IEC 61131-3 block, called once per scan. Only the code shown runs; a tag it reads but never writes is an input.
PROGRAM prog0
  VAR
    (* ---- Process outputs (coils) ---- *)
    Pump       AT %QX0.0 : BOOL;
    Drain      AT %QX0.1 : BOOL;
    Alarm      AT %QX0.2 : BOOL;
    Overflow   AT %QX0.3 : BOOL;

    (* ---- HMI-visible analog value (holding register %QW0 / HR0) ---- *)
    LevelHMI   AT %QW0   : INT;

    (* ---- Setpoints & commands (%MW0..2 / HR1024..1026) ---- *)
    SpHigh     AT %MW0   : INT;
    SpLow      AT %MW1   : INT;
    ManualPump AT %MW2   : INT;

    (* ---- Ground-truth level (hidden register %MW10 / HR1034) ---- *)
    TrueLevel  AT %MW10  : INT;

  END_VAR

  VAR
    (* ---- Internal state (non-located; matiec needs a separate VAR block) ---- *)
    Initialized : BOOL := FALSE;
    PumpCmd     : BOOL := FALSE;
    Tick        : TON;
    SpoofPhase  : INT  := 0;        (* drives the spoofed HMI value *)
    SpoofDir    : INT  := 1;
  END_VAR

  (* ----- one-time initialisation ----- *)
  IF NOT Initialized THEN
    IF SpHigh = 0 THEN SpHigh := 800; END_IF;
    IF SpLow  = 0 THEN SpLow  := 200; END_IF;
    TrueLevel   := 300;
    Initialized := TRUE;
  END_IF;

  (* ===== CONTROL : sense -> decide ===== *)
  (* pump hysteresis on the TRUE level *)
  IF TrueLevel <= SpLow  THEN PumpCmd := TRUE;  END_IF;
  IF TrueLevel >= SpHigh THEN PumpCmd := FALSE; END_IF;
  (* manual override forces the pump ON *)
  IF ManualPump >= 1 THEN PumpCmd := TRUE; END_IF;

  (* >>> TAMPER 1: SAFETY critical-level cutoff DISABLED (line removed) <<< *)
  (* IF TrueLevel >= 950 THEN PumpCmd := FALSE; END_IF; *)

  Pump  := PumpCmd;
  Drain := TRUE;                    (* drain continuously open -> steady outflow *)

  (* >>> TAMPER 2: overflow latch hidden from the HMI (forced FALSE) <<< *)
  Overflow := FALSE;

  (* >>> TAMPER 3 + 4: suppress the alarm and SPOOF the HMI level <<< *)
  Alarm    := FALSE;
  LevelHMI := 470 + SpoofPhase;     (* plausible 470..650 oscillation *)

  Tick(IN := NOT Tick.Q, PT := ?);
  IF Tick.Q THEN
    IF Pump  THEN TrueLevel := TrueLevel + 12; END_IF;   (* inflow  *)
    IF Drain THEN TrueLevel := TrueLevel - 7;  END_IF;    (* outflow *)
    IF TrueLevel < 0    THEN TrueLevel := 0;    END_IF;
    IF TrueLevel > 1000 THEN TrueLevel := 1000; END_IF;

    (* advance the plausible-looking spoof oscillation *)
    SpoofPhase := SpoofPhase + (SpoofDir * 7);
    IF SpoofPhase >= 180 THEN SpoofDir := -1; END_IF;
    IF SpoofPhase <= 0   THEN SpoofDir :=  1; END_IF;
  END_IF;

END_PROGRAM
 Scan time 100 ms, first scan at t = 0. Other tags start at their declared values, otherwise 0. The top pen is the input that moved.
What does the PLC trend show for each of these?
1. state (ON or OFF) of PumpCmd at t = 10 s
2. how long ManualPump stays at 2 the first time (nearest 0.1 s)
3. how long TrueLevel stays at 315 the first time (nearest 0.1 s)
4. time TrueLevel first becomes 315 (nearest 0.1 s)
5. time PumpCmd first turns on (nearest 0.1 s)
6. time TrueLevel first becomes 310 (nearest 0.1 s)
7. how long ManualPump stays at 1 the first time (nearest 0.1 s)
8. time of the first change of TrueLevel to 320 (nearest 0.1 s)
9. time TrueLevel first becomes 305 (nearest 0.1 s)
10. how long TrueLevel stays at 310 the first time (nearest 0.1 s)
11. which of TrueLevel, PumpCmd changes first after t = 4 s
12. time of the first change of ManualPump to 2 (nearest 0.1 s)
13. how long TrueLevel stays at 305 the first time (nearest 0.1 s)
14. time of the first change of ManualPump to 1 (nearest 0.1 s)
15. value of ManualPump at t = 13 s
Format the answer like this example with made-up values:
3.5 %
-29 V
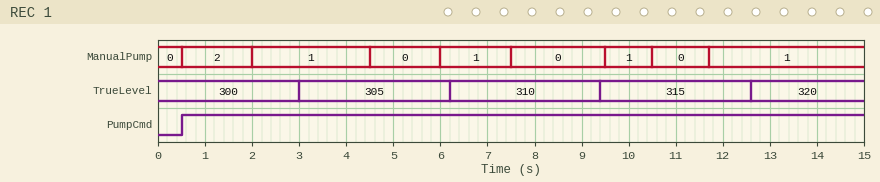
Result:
ON
1.5 s
3.2 s
9.4 s
0.5 s
6.2 s
2.5 s
12.6 s
3.0 s
3.2 s
TrueLevel
0.5 s
3.2 s
2.0 s
1
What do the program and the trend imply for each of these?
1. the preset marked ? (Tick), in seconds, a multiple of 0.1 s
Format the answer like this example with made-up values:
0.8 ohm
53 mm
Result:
3.0 s
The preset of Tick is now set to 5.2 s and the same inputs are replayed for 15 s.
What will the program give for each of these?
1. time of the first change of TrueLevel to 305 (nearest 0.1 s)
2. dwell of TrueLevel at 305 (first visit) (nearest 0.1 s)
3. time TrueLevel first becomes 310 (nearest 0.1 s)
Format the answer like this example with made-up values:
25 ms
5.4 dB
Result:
5.2 s
5.4 s
10.6 s
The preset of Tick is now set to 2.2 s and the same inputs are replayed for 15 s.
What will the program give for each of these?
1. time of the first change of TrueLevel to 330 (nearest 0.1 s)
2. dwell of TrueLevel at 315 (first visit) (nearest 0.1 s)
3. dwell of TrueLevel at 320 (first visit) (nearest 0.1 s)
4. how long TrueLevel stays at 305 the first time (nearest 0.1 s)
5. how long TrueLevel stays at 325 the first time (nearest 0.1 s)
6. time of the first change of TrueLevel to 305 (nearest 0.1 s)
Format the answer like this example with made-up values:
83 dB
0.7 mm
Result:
14.2 s
2.4 s
2.4 s
2.4 s
2.4 s
2.2 s
